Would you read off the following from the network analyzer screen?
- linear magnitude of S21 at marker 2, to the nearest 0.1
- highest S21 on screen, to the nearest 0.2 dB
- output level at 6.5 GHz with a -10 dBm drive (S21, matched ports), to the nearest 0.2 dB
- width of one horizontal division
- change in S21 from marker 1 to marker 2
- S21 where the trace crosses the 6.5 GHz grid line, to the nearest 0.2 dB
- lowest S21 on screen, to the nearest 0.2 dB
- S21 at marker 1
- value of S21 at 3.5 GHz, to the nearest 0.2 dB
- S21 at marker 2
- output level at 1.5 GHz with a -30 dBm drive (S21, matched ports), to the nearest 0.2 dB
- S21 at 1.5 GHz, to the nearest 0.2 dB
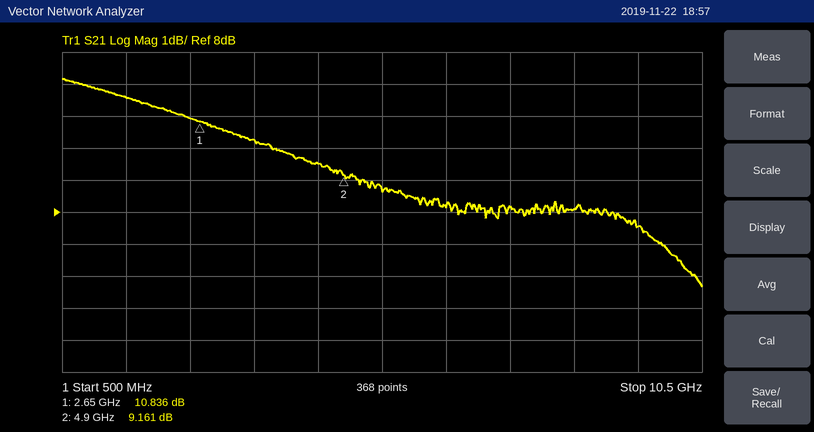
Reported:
2.9
12.2 dB
-1.8 dBm
1 GHz
-1.675 dB
8.2 dB
5.6 dB
10.836 dB
10.2 dB
9.161 dB
-18.4 dBm
11.6 dB
